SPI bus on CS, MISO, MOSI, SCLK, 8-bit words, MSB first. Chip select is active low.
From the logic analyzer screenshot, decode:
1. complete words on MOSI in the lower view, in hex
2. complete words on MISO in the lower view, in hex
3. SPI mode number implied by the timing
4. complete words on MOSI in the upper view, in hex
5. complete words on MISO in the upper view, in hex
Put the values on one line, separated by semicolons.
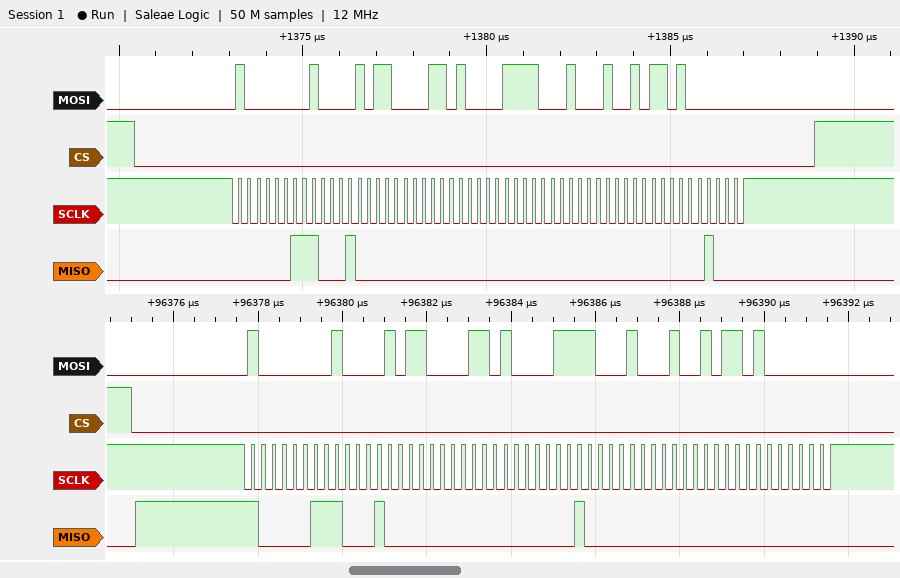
80, 85, 86, 87, 88, 96, 80; 83, 88, 00, 01, 00, 00, 00; 3; 80, 85, 86, 87, 88, 96, 80; 03, 88, 00, 00, 00, 00, 10
